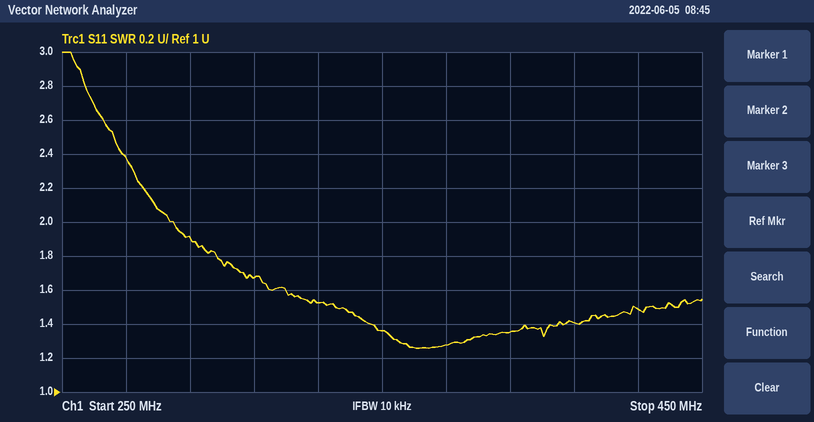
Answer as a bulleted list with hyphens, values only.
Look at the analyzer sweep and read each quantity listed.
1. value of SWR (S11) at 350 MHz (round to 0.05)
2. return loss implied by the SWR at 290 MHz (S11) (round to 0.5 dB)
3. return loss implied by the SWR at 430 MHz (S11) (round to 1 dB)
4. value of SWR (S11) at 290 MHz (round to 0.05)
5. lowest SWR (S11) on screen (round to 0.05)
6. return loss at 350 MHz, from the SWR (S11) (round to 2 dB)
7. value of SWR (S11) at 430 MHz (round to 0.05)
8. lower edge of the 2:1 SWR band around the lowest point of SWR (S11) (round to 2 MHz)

- 1.35
- 10.0 dB
- 14 dB
- 1.90
- 1.25
- 16 dB
- 1.50
- 284 MHz
